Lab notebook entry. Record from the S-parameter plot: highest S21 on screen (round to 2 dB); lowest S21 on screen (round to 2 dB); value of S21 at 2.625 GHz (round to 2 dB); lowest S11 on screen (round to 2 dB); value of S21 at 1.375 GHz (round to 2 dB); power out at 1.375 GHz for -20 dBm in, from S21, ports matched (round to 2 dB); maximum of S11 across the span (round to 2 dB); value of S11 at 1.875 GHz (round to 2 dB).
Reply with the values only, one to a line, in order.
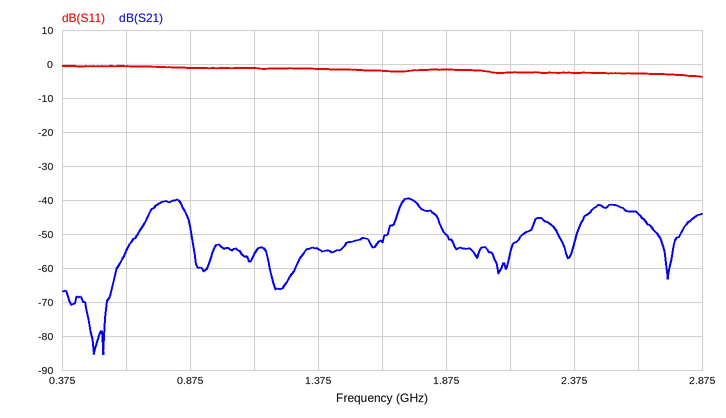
-40 dB
-86 dB
-44 dB
-4 dB
-54 dB
-74 dBm
0 dB
-2 dB
